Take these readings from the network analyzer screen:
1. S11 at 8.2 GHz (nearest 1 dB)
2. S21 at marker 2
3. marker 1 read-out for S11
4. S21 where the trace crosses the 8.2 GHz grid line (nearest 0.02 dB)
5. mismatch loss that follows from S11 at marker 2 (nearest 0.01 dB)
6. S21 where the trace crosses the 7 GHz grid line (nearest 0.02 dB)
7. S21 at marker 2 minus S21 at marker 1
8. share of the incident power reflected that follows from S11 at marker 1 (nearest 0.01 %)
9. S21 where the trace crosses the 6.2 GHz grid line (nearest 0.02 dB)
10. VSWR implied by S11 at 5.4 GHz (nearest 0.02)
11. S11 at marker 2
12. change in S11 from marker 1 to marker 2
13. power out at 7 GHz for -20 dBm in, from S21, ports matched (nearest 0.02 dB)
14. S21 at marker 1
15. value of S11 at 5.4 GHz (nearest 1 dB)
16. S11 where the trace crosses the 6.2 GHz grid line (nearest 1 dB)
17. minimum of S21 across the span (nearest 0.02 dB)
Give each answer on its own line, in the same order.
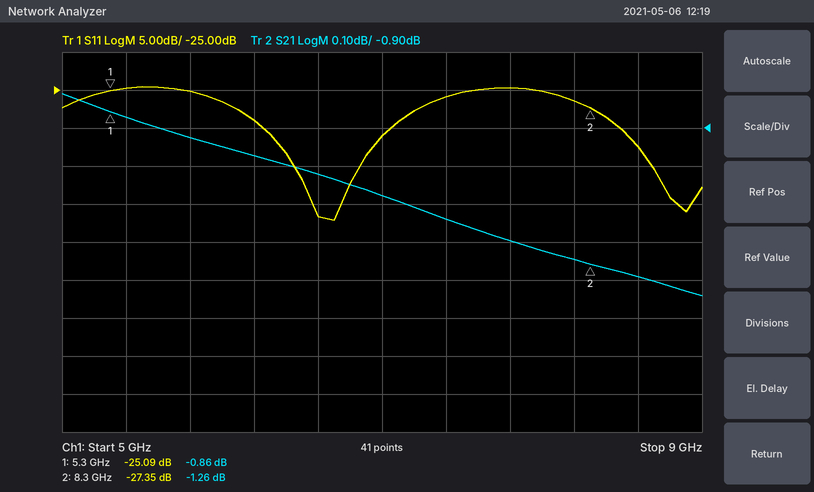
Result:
-26 dB
-1.26 dB
-25.09 dB
-1.24 dB
0.01 dB
-1.08 dB
-0.40 dB
0.31 %
-0.98 dB
1.12
-27.35 dB
-2.26 dB
-21.08 dBm
-0.86 dB
-25 dB
-29 dB
-1.34 dB
